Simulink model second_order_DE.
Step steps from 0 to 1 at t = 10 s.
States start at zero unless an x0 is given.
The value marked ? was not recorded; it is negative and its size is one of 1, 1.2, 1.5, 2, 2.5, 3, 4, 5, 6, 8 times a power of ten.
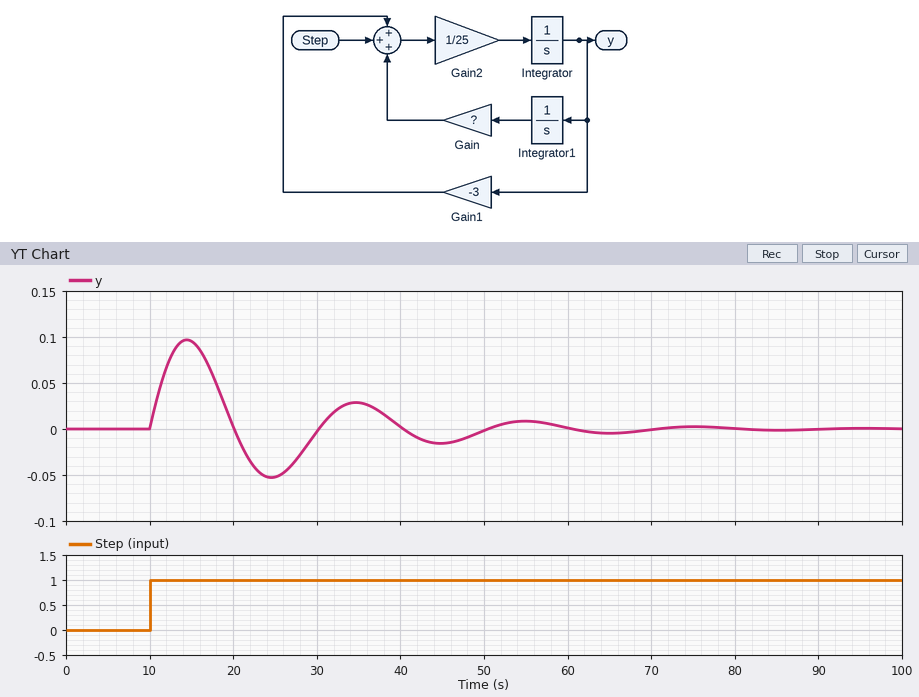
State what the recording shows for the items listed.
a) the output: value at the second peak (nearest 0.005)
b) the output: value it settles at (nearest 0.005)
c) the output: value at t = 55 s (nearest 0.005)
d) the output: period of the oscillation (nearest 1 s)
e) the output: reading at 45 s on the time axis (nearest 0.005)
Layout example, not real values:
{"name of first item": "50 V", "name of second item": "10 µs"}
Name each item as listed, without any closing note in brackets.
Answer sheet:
{"the output: value at the second peak": "0.030", "the output: value it settles at": "0.000", "the output: value at t = 55 s": "0.010", "the output: period of the oscillation": "20 s", "the output: reading at 45 s on the time axis": "-0.015"}
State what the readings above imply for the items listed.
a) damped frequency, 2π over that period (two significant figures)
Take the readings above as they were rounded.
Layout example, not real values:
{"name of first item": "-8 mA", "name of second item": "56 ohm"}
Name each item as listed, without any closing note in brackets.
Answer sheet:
{"damped frequency, 2π over that period": "0.31 rad/s"}
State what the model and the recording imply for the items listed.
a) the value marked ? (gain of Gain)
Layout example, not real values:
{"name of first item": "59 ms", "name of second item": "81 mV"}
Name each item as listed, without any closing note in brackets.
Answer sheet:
{"the value marked ?": "-2.5"}
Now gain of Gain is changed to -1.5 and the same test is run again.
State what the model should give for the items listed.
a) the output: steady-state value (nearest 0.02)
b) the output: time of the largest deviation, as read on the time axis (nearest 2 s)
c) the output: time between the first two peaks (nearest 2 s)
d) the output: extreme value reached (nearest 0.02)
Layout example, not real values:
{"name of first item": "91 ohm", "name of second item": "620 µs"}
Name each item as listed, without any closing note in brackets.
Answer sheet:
{"the output: steady-state value": "0.00", "the output: time of the largest deviation, as read on the time axis": "16 s", "the output: time between the first two peaks": "26 s", "the output: extreme value reached": "0.12"}
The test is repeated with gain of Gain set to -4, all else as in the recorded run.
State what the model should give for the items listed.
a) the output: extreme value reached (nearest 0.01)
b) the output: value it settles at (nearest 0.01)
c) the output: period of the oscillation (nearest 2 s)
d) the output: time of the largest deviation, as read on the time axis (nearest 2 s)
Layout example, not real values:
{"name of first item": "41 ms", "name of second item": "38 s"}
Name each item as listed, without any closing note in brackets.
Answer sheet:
{"the output: extreme value reached": "0.08", "the output: value it settles at": "0.00", "the output: period of the oscillation": "16 s", "the output: time of the largest deviation, as read on the time axis": "14 s"}
